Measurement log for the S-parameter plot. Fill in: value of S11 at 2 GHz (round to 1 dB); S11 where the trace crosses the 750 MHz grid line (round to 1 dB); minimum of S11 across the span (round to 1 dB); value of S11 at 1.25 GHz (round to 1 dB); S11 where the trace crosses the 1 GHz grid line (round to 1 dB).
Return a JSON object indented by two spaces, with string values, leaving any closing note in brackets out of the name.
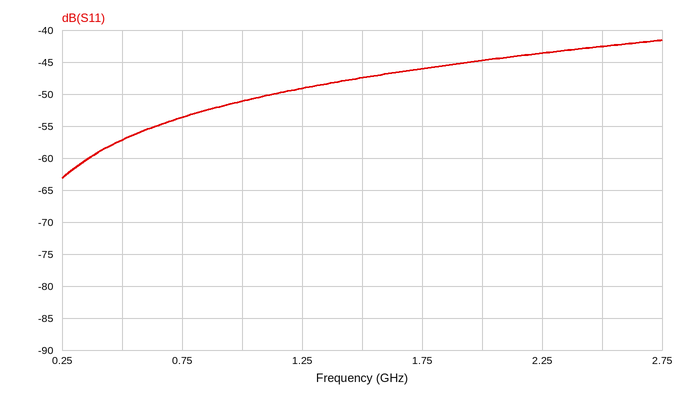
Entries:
{
  "value of S11 at 2 GHz": "-45 dB",
  "S11 where the trace crosses the 750 MHz grid line": "-54 dB",
  "minimum of S11 across the span": "-63 dB",
  "value of S11 at 1.25 GHz": "-49 dB",
  "S11 where the trace crosses the 1 GHz grid line": "-51 dB"
}
